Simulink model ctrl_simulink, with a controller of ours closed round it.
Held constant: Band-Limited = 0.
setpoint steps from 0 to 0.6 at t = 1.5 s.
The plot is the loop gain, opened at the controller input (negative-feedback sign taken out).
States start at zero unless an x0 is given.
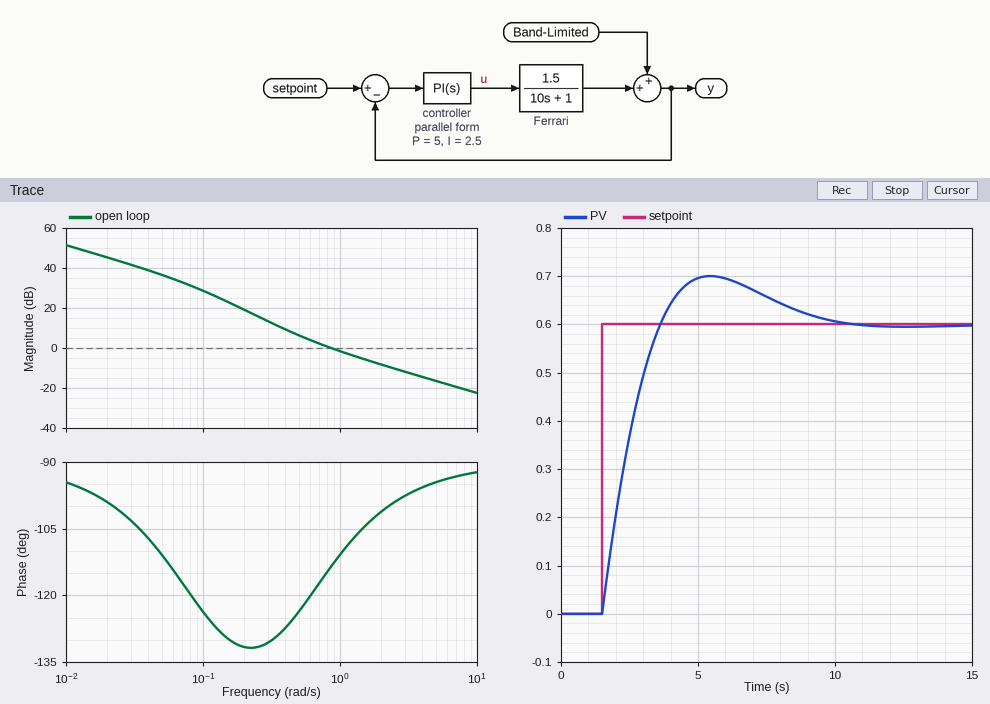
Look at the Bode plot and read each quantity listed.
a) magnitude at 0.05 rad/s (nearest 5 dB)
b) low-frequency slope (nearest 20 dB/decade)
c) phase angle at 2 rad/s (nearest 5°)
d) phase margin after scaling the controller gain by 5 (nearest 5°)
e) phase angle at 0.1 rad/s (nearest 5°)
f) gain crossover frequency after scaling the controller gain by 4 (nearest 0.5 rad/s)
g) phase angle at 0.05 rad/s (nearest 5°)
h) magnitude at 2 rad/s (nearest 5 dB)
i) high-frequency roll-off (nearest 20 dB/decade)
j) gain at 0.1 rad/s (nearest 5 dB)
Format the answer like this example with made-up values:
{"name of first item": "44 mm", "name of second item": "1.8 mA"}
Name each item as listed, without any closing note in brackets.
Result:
{"magnitude at 0.05 rad/s": "35 dB", "low-frequency slope": "-20 dB/decade", "phase angle at 2 rad/s": "-100°", "phase margin after scaling the controller gain by 5": "85°", "phase angle at 0.1 rad/s": "-125°", "gain crossover frequency after scaling the controller gain by 4": "3.0 rad/s", "phase angle at 0.05 rad/s": "-110°", "magnitude at 2 rad/s": "-10 dB", "high-frequency roll-off": "-20 dB/decade", "gain at 0.1 rad/s": "30 dB"}
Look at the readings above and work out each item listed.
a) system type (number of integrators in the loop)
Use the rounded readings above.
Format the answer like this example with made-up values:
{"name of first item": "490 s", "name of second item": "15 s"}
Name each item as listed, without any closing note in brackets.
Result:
{"system type": "1"}
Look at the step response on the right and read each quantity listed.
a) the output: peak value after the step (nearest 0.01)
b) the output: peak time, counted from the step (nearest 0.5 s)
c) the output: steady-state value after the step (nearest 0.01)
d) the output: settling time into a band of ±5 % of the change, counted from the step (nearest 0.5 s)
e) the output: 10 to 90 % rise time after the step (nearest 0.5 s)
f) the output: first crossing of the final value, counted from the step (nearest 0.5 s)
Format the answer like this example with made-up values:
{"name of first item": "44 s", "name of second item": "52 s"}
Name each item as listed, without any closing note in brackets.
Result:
{"the output: peak value after the step": "0.70", "the output: peak time, counted from the step": "4.0 s", "the output: steady-state value after the step": "0.60", "the output: settling time into a band of ±5 % of the change, counted from the step": "7.0 s", "the output: 10 to 90 % rise time after the step": "1.5 s", "the output: first crossing of the final value, counted from the step": "2.0 s"}
